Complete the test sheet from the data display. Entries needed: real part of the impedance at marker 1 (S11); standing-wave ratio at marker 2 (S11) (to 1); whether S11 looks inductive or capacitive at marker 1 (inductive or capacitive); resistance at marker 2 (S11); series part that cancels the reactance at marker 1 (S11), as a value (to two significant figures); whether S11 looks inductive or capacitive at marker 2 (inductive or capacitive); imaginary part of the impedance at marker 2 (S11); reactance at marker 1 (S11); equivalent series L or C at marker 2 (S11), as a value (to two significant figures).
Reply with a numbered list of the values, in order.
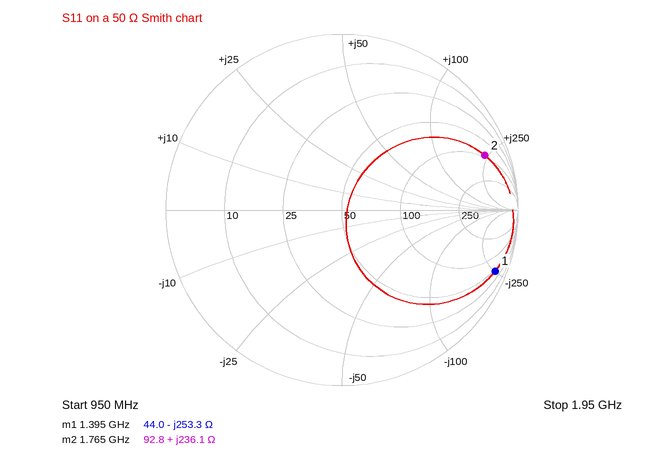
1. 44.0 Ω
2. 14
3. capacitive
4. 92.8 Ω
5. 29 nH
6. inductive
7. +236.1 Ω
8. -253.3 Ω
9. 21 nH
